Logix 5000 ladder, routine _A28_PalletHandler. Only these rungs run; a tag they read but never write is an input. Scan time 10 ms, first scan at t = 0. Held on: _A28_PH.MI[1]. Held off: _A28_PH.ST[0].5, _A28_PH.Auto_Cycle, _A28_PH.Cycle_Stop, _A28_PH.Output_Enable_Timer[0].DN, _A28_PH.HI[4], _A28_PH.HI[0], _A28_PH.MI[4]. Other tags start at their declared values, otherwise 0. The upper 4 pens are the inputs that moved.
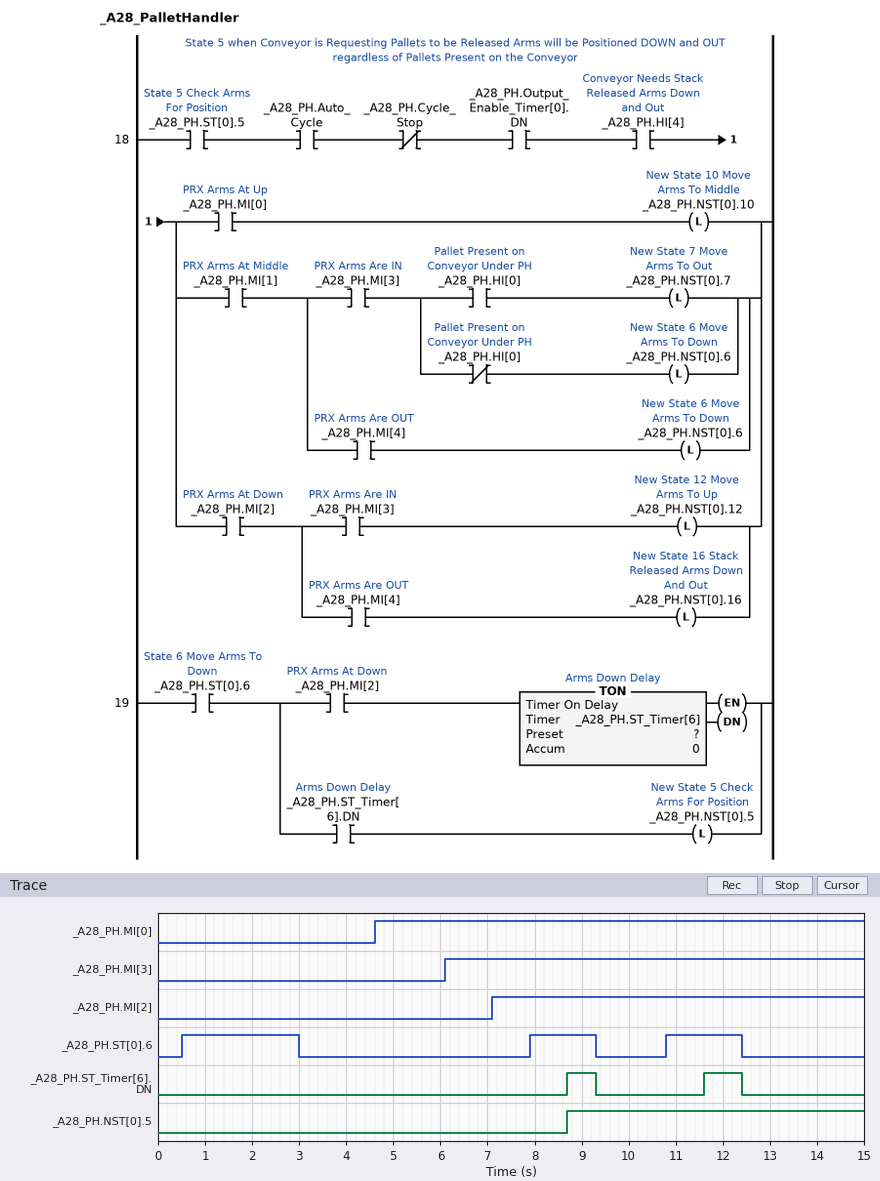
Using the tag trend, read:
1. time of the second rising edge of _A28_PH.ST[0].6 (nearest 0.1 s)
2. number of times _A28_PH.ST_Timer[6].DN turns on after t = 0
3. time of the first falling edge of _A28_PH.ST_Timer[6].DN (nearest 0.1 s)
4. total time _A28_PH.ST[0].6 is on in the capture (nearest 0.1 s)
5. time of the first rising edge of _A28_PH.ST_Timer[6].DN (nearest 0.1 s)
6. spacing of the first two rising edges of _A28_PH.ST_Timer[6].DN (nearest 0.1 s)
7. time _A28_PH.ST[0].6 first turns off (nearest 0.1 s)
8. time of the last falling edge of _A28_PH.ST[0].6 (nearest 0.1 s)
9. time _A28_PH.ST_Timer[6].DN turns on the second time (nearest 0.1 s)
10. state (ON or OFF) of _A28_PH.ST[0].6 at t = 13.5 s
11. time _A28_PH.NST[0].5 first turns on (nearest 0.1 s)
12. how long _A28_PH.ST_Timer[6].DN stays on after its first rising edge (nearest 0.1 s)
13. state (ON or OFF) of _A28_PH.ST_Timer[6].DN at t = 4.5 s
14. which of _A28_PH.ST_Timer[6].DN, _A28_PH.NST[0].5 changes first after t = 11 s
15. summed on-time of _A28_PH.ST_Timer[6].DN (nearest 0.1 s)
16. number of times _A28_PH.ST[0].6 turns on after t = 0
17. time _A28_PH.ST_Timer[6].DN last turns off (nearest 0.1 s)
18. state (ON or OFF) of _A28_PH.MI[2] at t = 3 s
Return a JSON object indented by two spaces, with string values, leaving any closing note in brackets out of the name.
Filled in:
{
  "time of the second rising edge of _A28_PH.ST[0].6": "7.9 s",
  "number of times _A28_PH.ST_Timer[6].DN turns on after t = 0": "2",
  "time of the first falling edge of _A28_PH.ST_Timer[6].DN": "9.3 s",
  "total time _A28_PH.ST[0].6 is on in the capture": "5.5 s",
  "time of the first rising edge of _A28_PH.ST_Timer[6].DN": "8.7 s",
  "spacing of the first two rising edges of _A28_PH.ST_Timer[6].DN": "2.9 s",
  "time _A28_PH.ST[0].6 first turns off": "3.0 s",
  "time of the last falling edge of _A28_PH.ST[0].6": "12.4 s",
  "time _A28_PH.ST_Timer[6].DN turns on the second time": "11.6 s",
  "state (ON or OFF) of _A28_PH.ST[0].6 at t = 13.5 s": "OFF",
  "time _A28_PH.NST[0].5 first turns on": "8.7 s",
  "how long _A28_PH.ST_Timer[6].DN stays on after its first rising edge": "0.6 s",
  "state (ON or OFF) of _A28_PH.ST_Timer[6].DN at t = 4.5 s": "OFF",
  "which of _A28_PH.ST_Timer[6].DN, _A28_PH.NST[0].5 changes first after t = 11 s": "_A28_PH.ST_Timer[6].DN",
  "summed on-time of _A28_PH.ST_Timer[6].DN": "1.4 s",
  "number of times _A28_PH.ST[0].6 turns on after t = 0": "3",
  "time _A28_PH.ST_Timer[6].DN last turns off": "12.4 s",
  "state (ON or OFF) of _A28_PH.MI[2] at t = 3 s": "OFF"
}
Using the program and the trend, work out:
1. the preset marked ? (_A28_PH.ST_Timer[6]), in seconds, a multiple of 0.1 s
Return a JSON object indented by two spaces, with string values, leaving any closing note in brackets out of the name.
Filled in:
{
  "the preset marked ? (_A28_PH.ST_Timer[6]), in seconds, a multiple of 0.1 s": "0.8 s"
}
